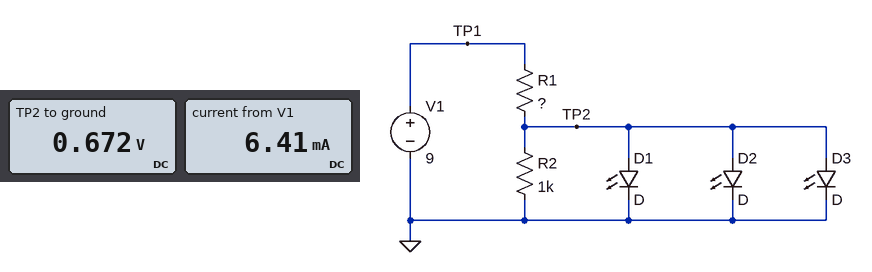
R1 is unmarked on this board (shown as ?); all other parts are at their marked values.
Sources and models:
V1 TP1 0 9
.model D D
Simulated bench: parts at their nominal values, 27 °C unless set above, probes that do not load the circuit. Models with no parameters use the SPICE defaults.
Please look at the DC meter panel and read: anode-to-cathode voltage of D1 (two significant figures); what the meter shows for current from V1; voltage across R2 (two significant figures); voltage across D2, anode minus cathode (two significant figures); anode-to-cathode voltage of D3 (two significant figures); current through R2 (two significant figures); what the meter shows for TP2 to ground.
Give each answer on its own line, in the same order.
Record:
670 mV
6.41 mA
670 mV
670 mV
670 mV
670 µA
0.672 V
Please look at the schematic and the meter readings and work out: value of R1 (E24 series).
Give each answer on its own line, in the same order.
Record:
1.3 kΩ
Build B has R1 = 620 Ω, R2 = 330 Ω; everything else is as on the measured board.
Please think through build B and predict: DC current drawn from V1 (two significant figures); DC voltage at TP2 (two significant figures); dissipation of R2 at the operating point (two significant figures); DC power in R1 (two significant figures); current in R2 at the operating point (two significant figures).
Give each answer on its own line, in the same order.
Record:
13 mA
690 mV
1.4 mW
110 mW
2.1 mA
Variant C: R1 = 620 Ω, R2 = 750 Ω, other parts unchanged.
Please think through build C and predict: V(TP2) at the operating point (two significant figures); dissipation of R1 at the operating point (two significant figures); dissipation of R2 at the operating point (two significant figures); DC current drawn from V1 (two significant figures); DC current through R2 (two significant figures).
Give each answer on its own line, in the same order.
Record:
690 mV
110 mW
640 µW
13 mA
920 µA
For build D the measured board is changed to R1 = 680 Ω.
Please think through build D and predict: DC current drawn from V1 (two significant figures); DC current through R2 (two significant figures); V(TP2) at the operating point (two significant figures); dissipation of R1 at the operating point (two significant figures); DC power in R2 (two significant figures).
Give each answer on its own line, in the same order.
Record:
12 mA
690 µA
690 mV
100 mW
480 µW
